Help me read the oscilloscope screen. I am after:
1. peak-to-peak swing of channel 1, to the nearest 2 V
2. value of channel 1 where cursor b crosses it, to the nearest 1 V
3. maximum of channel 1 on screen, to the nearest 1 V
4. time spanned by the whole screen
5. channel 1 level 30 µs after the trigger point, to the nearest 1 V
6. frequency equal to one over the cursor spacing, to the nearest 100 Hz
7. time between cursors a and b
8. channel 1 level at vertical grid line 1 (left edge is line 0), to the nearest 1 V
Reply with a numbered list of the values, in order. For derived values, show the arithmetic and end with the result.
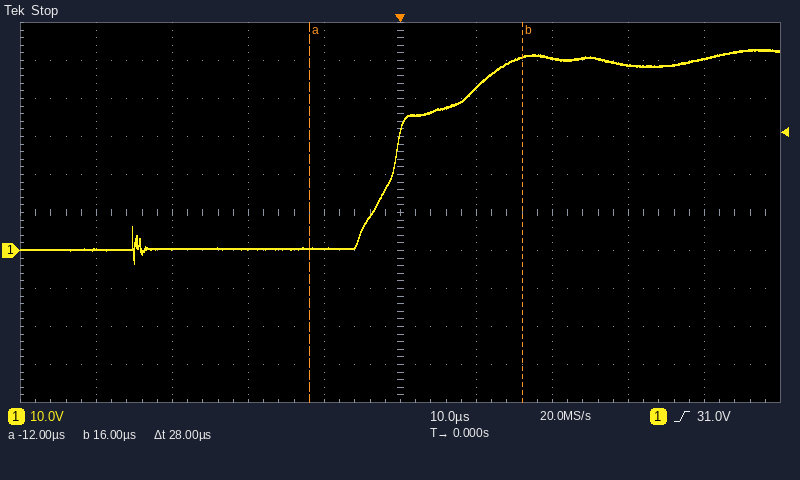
1. 56 V
2. 51 V
3. 53 V
4. 100 µs
5. 49 V
6. 1 / 28 µs ≈ 35.7 kHz
7. 28 µs
8. 0 V
